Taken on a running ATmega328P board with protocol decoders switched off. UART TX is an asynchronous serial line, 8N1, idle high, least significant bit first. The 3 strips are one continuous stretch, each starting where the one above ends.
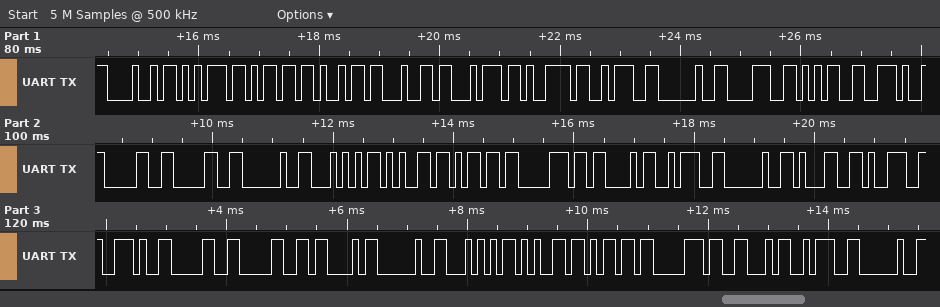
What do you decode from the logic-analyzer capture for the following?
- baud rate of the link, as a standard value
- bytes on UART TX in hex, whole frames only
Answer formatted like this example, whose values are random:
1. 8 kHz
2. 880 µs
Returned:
1. 9600 baud
2. 48 75 6D 69 64 74 79 3A 20 38 35 2E 30 30 20 54 65 6D 70 43 3A 20 31 39 2E 30 30 43 20 54 65 6D 70 46 3A 20
